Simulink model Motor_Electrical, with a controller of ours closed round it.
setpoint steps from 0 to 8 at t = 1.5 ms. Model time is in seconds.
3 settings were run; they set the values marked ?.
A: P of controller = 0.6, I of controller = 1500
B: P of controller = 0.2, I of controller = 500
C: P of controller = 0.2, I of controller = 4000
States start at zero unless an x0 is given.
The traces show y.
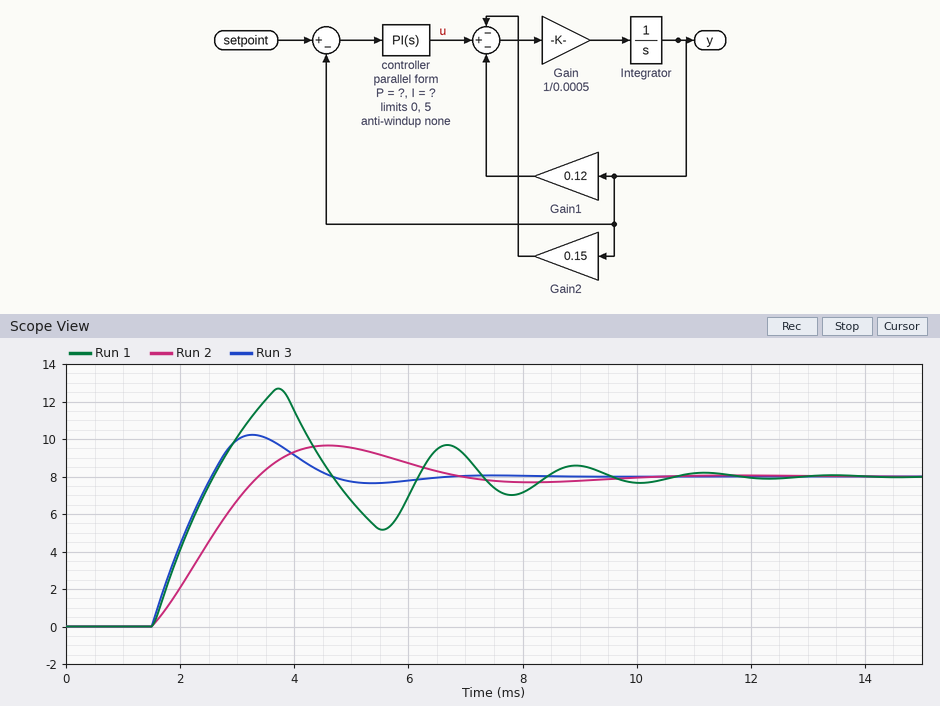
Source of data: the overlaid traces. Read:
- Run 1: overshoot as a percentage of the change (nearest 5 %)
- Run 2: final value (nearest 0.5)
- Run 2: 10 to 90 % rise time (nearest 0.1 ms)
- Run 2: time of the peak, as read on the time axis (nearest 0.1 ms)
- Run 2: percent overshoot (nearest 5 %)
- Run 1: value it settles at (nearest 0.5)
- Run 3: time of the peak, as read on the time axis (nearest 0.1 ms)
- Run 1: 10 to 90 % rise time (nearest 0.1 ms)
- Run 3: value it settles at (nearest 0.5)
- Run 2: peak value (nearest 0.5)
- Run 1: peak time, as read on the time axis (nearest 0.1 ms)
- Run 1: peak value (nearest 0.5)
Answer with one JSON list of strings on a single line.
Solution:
["60 %", "8.0", "1.4 ms", "4.6 ms", "20 %", "8.0", "3.3 ms", "0.8 ms", "8.0", "9.5", "3.7 ms", "12.5"]
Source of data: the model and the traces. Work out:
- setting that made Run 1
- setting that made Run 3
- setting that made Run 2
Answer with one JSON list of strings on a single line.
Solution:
["C", "A", "B"]
